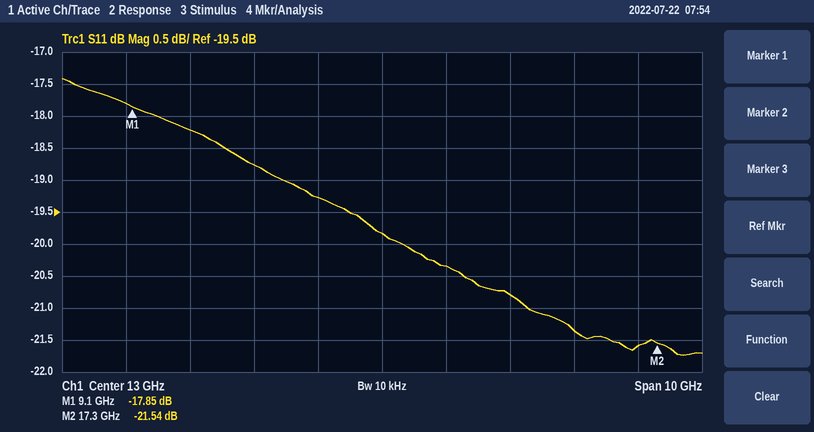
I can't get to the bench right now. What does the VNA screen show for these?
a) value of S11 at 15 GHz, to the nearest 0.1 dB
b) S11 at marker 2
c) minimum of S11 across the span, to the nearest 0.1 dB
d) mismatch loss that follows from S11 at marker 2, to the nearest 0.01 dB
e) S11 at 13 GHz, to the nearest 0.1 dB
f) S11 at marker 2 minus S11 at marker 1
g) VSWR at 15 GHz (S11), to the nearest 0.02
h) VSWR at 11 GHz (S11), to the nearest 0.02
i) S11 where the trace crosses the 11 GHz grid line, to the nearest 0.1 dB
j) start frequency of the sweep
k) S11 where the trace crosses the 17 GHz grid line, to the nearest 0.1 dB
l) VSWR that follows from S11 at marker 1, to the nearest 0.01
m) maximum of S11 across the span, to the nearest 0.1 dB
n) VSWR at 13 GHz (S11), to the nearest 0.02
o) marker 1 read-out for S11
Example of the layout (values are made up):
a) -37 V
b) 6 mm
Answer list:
a) -20.8 dB
b) -21.54 dB
c) -21.7 dB
d) 0.03 dB
e) -19.8 dB
f) -3.69 dB
g) 1.20
h) 1.26
i) -18.8 dB
j) 8 GHz
k) -21.6 dB
l) 1.29
m) -17.4 dB
n) 1.22
o) -17.85 dB
